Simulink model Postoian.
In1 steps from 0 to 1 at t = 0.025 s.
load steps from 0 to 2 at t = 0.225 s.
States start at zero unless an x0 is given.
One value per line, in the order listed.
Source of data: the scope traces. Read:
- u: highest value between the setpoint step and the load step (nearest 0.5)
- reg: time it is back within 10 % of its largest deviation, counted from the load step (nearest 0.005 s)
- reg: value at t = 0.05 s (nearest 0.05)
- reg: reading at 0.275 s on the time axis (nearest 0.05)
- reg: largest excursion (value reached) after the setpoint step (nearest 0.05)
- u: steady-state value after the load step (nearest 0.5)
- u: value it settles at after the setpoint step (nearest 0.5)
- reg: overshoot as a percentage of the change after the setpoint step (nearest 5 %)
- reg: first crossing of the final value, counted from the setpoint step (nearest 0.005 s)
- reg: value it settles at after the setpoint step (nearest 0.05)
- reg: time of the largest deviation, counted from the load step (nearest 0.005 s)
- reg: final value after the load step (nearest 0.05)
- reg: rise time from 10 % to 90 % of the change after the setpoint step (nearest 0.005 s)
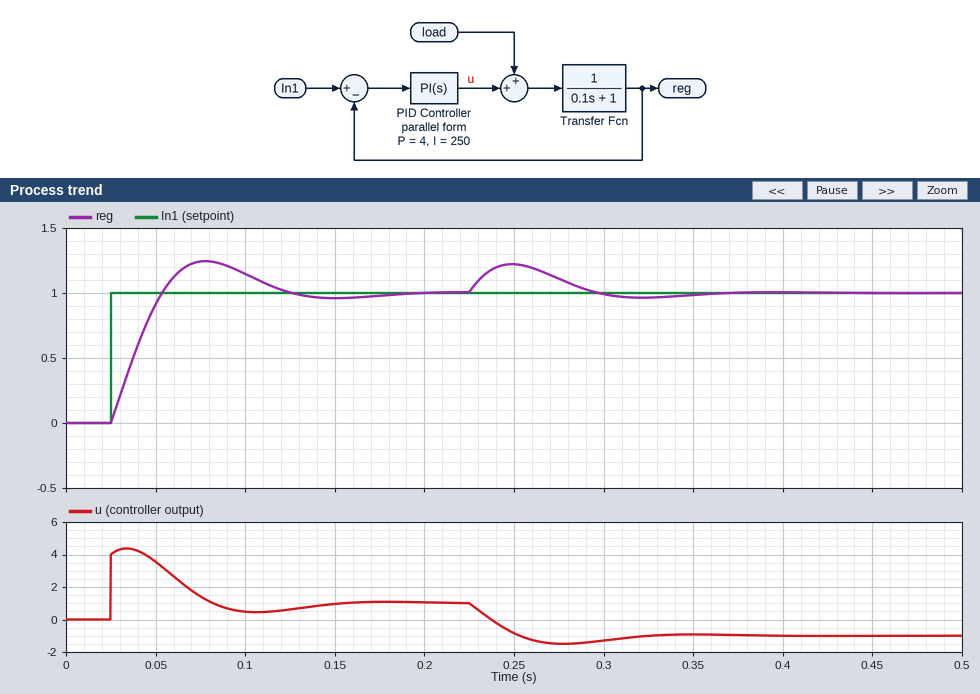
4.5
0.120 s
0.90
1.10
1.25
-1.0
1.0
25 %
0.030 s
1.00
0.025 s
1.00
0.020 s
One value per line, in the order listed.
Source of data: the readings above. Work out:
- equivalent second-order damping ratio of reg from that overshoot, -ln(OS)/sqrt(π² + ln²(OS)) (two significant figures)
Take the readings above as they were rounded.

0.40
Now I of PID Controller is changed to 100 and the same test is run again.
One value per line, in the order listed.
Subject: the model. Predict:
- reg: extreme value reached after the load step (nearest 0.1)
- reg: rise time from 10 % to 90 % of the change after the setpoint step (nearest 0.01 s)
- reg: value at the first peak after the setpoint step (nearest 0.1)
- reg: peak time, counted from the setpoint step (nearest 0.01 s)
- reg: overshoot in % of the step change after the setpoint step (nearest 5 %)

1.3
0.03 s
1.1
0.08 s
10 %
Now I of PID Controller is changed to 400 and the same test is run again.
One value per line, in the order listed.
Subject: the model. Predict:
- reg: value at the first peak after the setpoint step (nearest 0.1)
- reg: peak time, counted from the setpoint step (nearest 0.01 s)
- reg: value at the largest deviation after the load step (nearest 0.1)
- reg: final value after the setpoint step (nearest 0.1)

1.3
0.04 s
1.2
1.0
